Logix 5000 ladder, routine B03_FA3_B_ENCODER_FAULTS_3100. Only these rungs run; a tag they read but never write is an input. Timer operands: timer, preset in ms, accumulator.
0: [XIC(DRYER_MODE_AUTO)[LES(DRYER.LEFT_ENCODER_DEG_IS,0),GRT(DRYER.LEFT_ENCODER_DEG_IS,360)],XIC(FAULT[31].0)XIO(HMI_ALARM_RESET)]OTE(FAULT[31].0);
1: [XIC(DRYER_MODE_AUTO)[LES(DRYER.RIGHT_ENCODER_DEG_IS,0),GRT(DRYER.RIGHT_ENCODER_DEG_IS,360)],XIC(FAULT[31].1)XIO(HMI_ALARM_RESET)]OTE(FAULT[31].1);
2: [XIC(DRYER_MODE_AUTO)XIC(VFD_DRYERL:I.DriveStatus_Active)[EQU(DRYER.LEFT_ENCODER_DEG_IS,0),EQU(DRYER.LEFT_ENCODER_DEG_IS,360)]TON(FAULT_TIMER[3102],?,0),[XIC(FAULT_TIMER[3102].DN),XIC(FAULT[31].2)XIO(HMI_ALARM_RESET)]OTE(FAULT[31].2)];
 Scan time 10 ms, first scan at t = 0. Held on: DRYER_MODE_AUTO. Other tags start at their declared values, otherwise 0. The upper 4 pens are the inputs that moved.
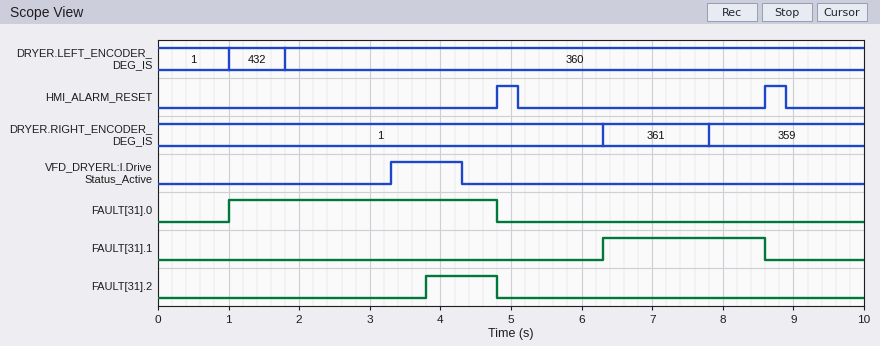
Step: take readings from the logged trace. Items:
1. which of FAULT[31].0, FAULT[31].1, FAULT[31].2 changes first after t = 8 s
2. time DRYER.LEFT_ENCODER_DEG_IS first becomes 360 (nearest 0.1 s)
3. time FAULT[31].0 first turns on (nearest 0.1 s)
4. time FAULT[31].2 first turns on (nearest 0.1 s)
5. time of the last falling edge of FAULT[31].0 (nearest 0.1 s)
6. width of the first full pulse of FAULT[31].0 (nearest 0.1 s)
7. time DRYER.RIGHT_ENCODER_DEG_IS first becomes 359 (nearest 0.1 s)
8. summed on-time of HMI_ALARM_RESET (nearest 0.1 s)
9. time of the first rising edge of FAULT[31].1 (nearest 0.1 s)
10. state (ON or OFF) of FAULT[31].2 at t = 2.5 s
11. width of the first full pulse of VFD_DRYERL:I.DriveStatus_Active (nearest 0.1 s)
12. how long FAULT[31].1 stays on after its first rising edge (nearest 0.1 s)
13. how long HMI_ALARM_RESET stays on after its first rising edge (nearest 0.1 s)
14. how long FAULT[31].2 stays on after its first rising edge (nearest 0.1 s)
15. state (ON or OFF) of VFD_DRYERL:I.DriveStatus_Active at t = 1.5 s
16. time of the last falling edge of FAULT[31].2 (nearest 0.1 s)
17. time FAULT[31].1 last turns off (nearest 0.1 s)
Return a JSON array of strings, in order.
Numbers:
["FAULT[31].1", "1.8 s", "1.0 s", "3.8 s", "4.8 s", "3.8 s", "7.8 s", "0.6 s", "6.3 s", "OFF", "1.0 s", "2.3 s", "0.3 s", "1.0 s", "OFF", "4.8 s", "8.6 s"]
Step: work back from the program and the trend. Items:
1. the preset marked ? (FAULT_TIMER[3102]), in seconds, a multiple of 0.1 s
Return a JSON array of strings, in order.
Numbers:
["0.5 s"]
